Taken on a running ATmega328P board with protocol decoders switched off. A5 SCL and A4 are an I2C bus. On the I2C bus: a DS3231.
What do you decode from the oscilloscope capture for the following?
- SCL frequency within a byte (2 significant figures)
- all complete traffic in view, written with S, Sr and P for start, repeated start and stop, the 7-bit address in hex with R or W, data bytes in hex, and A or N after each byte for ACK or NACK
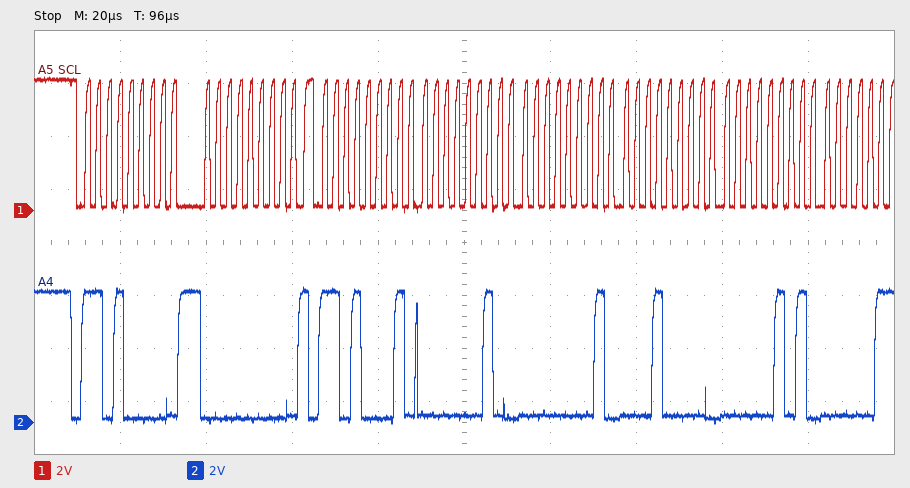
400 kHz
S 68W A 00 A Sr 68R A 02 A 01 A 10 A 05 A
